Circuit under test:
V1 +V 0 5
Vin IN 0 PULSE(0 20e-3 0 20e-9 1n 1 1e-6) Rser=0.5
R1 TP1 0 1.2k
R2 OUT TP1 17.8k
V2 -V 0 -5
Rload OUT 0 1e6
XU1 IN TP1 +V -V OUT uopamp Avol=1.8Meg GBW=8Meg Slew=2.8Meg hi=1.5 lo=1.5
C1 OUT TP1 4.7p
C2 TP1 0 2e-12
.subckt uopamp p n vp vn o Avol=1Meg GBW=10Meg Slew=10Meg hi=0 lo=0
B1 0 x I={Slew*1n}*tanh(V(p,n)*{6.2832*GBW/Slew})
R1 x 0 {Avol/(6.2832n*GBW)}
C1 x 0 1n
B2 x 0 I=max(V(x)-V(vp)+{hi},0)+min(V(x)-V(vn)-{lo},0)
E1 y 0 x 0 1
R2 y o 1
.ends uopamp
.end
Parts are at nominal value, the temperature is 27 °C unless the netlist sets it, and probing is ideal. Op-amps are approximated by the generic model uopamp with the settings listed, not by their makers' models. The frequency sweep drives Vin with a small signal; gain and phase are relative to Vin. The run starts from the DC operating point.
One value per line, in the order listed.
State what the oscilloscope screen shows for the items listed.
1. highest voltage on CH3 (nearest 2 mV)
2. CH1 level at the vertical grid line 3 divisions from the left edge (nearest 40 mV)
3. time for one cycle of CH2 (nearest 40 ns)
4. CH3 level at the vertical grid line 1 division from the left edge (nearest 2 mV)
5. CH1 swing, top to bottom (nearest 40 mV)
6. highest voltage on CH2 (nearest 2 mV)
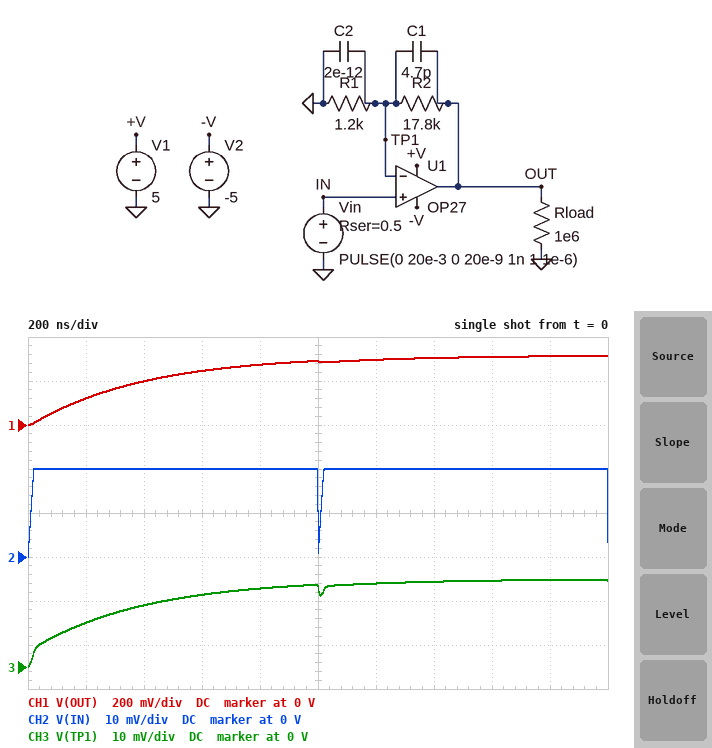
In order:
20 mV
240 mV
1.00 µs
10 mV
320 mV
20 mV
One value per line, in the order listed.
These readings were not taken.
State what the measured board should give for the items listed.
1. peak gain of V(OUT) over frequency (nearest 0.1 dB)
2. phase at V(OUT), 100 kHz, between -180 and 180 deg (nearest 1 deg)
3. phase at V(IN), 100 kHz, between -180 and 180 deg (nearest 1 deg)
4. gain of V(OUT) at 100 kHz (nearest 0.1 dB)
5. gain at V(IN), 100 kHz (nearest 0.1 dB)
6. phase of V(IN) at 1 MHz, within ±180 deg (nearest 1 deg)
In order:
24.0 dB
-14 deg
0 deg
23.7 dB
0 dB
0 deg
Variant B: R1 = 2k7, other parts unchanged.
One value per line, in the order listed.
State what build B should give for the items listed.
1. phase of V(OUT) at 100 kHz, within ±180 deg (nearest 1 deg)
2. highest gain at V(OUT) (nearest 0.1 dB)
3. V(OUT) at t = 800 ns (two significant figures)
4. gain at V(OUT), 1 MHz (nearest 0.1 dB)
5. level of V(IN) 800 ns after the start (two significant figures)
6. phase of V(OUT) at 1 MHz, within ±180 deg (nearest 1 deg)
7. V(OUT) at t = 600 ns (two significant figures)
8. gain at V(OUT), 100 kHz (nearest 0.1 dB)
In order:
-8 deg
17.6 dB
150 mV
12.9 dB
20 mV
-53 deg
140 mV
17.5 dB
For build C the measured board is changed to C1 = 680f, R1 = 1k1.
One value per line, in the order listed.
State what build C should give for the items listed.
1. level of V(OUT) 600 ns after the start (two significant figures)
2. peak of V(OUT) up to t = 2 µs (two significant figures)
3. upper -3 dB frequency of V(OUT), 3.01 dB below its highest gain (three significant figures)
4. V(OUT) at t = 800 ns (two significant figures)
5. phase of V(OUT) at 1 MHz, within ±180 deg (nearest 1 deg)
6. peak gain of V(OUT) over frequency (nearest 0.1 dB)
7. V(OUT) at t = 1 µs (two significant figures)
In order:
280 mV
340 mV
453 kHz
310 mV
-66 deg
24.7 dB
320 mV
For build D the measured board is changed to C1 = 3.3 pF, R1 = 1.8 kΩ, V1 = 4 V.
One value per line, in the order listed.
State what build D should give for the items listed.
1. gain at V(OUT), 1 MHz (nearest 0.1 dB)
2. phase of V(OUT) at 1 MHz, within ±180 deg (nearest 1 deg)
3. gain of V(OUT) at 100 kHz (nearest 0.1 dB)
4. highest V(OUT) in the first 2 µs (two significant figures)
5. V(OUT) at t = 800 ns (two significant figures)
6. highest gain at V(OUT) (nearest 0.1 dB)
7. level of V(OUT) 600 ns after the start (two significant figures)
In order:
14.9 dB
-59 deg
20.6 dB
220 mV
210 mV
20.7 dB
190 mV
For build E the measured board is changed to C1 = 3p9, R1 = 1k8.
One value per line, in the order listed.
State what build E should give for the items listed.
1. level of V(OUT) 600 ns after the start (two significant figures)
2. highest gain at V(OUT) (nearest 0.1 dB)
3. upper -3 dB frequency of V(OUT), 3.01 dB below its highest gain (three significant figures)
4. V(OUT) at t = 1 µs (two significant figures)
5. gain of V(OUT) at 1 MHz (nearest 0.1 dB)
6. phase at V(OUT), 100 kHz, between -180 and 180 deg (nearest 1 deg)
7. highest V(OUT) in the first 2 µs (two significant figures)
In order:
190 mV
20.7 dB
572 kHz
210 mV
14.7 dB
-10 deg
220 mV
